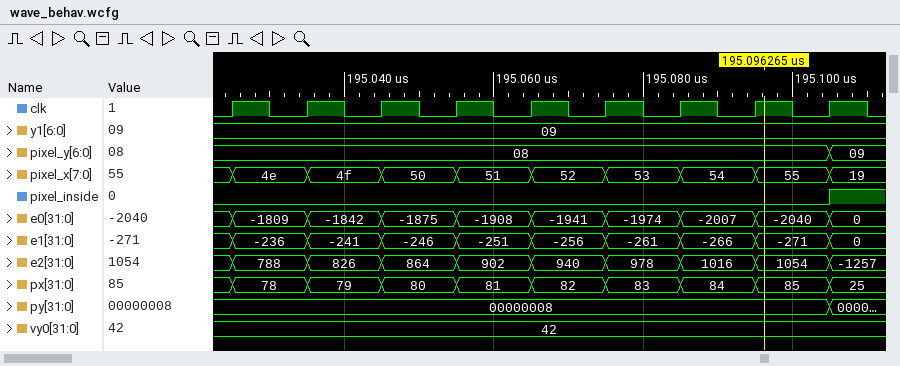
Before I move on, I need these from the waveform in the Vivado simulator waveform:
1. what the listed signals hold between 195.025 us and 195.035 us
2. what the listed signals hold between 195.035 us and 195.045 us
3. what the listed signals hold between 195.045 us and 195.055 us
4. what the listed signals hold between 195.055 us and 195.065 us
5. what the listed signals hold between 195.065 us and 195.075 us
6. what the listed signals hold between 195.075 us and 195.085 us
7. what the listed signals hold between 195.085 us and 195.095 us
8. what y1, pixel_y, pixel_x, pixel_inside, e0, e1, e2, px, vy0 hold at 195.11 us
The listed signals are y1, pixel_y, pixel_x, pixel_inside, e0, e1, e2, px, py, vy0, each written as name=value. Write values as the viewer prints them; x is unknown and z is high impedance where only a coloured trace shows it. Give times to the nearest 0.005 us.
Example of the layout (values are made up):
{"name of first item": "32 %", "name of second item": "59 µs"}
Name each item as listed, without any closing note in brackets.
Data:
{"what the listed signals hold between 195.025 us and 195.035 us": "y1=09, pixel_y=08, pixel_x=4e, pixel_inside=0, e0=-1809, e1=-236, e2=788, px=78, py=00000008, vy0=42", "what the listed signals hold between 195.035 us and 195.045 us": "y1=09, pixel_y=08, pixel_x=4f, pixel_inside=0, e0=-1842, e1=-241, e2=826, px=79, py=00000008, vy0=42", "what the listed signals hold between 195.045 us and 195.055 us": "y1=09, pixel_y=08, pixel_x=50, pixel_inside=0, e0=-1875, e1=-246, e2=864, px=80, py=00000008, vy0=42", "what the listed signals hold between 195.055 us and 195.065 us": "y1=09, pixel_y=08, pixel_x=51, pixel_inside=0, e0=-1908, e1=-251, e2=902, px=81, py=00000008, vy0=42", "what the listed signals hold between 195.065 us and 195.075 us": "y1=09, pixel_y=08, pixel_x=52, pixel_inside=0, e0=-1941, e1=-256, e2=940, px=82, py=00000008, vy0=42", "what the listed signals hold between 195.075 us and 195.085 us": "y1=09, pixel_y=08, pixel_x=53, pixel_inside=0, e0=-1974, e1=-261, e2=978, px=83, py=00000008, vy0=42", "what the listed signals hold between 195.085 us and 195.095 us": "y1=09, pixel_y=08, pixel_x=54, pixel_inside=0, e0=-2007, e1=-266, e2=1016, px=84, py=00000008, vy0=42", "what y1, pixel_y, pixel_x, pixel_inside, e0, e1, e2, px, vy0 hold at 195.11 us": "y1=09, pixel_y=09, pixel_x=19, pixel_inside=1, e0=0, e1=0, e2=-1257, px=25, vy0=42"}
